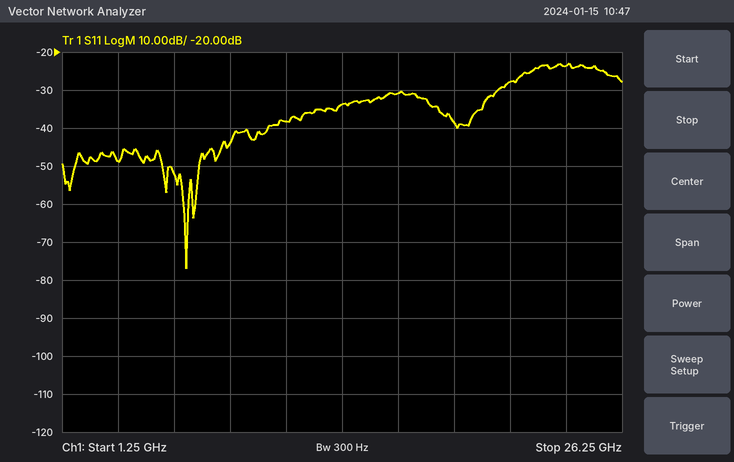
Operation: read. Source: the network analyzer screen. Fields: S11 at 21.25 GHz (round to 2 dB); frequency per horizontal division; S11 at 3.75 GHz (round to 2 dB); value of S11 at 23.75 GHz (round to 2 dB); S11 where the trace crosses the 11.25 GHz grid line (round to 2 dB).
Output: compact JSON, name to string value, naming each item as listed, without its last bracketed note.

{"S11 at 21.25 GHz": "-28 dB", "frequency per horizontal division": "2.5 GHz", "S11 at 3.75 GHz": "-48 dB", "value of S11 at 23.75 GHz": "-24 dB", "S11 where the trace crosses the 11.25 GHz grid line": "-38 dB"}
